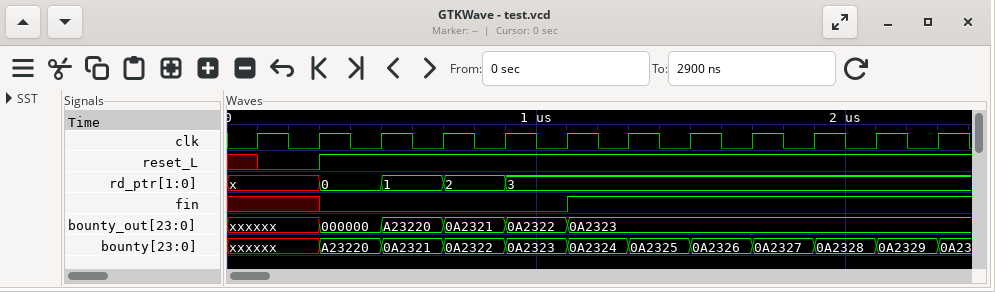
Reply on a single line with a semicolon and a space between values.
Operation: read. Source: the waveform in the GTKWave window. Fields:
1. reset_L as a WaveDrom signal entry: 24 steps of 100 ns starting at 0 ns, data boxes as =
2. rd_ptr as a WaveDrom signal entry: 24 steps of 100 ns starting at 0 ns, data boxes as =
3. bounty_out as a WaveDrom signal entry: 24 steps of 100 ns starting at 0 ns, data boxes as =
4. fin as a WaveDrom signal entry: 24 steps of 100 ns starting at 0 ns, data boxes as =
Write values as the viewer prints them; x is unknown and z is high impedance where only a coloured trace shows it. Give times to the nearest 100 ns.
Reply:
{name: 'reset_L', wave: 'x0.1....................'}; {name: 'rd_ptr', wave: 'x..=.=.=.=..............', data: '0 1 2 3'}; {name: 'bounty_out', wave: 'x..=.=.=.=.=............', data: '000000 A23220 0A2321 0A2322 0A2323'}; {name: 'fin', wave: 'x..0.......1............'}
